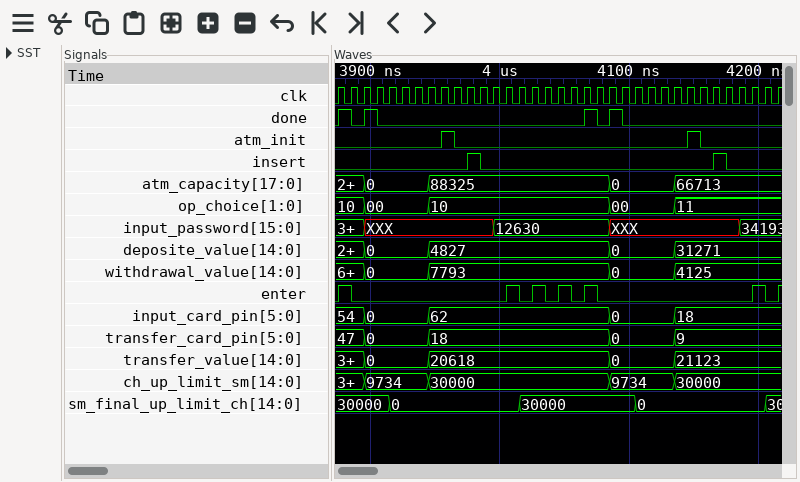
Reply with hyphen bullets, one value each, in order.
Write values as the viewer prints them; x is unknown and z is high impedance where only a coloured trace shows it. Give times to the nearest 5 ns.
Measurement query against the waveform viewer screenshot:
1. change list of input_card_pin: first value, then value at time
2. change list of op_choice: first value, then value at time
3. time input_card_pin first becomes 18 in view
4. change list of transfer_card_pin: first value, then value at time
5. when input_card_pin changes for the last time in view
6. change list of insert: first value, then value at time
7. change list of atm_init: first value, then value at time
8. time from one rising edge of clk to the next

- 54, 0 at 3895 ns, 62 at 3945 ns, 0 at 4085 ns, 18 at 4135 ns
- 10, 00 at 3895 ns, 10 at 3945 ns, 00 at 4085 ns, 11 at 4135 ns
- 4135 ns
- 47, 0 at 3895 ns, 18 at 3945 ns, 0 at 4085 ns, 9 at 4135 ns
- 4135 ns
- 0, 1 at 3975 ns, 0 at 3985 ns, 1 at 4165 ns, 0 at 4175 ns
- 0, 1 at 3955 ns, 0 at 3965 ns, 1 at 4145 ns, 0 at 4155 ns
- 10 ns
